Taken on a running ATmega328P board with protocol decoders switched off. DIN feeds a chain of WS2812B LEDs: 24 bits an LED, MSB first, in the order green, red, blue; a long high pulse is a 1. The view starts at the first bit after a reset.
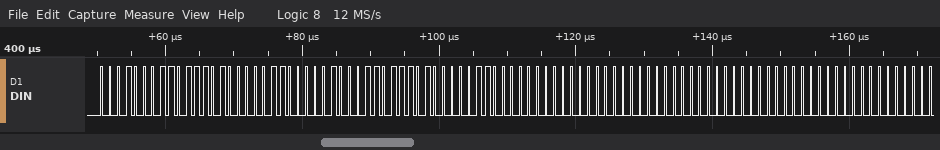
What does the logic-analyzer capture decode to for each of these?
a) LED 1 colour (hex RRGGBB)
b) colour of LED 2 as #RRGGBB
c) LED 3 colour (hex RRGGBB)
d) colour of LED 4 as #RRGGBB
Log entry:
#BA110C
#BA110C
#000000
#000000
